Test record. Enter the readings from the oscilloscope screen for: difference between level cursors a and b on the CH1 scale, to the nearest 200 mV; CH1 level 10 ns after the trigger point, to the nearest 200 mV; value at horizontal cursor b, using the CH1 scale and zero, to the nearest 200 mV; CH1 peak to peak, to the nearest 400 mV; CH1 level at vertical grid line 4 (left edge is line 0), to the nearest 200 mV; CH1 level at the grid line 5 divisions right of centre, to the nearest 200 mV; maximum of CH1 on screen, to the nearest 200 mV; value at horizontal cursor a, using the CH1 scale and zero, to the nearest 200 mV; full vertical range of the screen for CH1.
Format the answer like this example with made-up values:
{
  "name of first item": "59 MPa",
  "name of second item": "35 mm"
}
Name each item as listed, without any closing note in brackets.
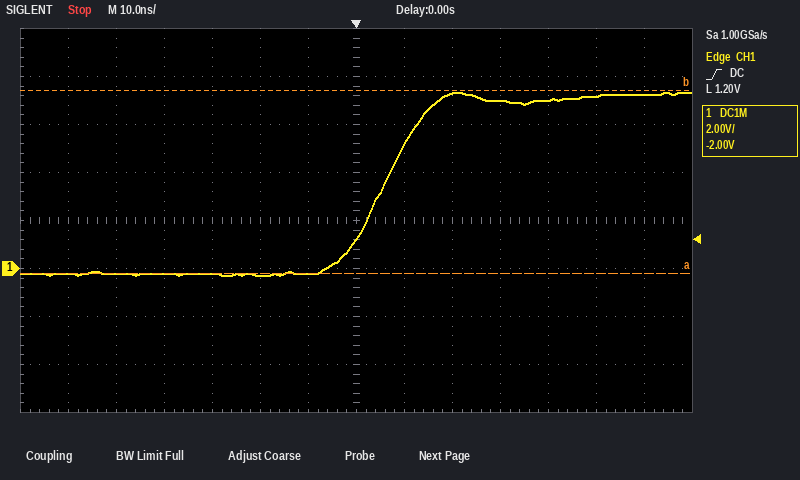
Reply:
{
  "difference between level cursors a and b on the CH1 scale, to the nearest 200 mV": "7.6 V",
  "CH1 level 10 ns after the trigger point, to the nearest 200 mV": "5.2 V",
  "value at horizontal cursor b, using the CH1 scale and zero, to the nearest 200 mV": "7.4 V",
  "CH1 peak to peak, to the nearest 400 mV": "7.6 V",
  "CH1 level at vertical grid line 4 (left edge is line 0), to the nearest 200 mV": "-200 mV",
  "CH1 level at the grid line 5 divisions right of centre, to the nearest 200 mV": "7.2 V",
  "maximum of CH1 on screen, to the nearest 200 mV": "7.4 V",
  "value at horizontal cursor a, using the CH1 scale and zero, to the nearest 200 mV": "-200 mV",
  "full vertical range of the screen for CH1": "16 V"
}
